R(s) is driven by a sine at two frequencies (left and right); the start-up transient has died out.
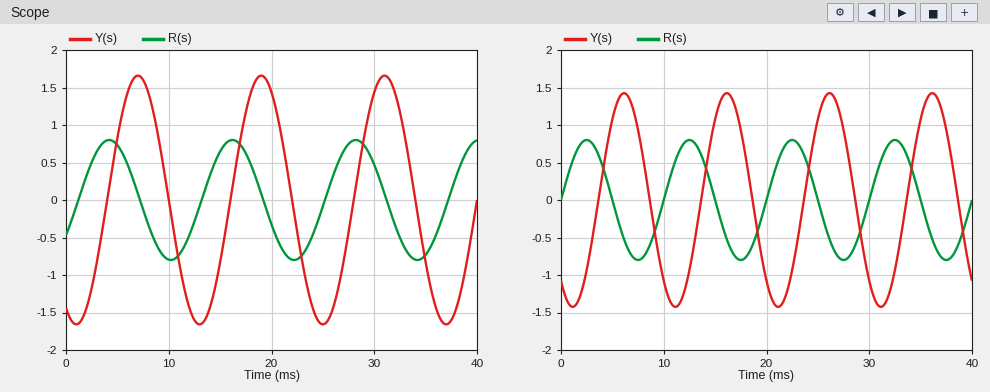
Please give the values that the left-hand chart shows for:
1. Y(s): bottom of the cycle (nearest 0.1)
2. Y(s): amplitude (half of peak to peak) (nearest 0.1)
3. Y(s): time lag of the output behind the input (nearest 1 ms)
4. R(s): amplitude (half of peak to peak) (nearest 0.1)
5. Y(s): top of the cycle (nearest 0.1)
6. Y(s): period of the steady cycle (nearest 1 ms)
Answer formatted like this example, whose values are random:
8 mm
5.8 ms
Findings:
-1.7
1.7
3 ms
0.8
1.7
12 ms
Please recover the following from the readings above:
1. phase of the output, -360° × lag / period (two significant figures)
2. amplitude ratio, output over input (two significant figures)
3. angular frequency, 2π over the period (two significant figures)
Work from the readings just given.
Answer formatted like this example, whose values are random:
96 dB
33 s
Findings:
-90°
2.1
0.52 rad/ms
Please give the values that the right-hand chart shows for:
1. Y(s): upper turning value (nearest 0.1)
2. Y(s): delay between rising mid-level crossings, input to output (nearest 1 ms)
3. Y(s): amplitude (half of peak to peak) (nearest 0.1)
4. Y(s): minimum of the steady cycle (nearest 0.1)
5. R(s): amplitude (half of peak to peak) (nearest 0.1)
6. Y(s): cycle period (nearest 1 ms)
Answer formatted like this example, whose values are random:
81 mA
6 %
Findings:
1.4
4 ms
1.4
-1.4
0.8
10 ms
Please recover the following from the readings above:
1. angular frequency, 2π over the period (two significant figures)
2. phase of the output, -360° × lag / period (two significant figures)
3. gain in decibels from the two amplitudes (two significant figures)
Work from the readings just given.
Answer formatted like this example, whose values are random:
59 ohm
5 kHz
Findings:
0.63 rad/ms
-140°
4.9 dB
